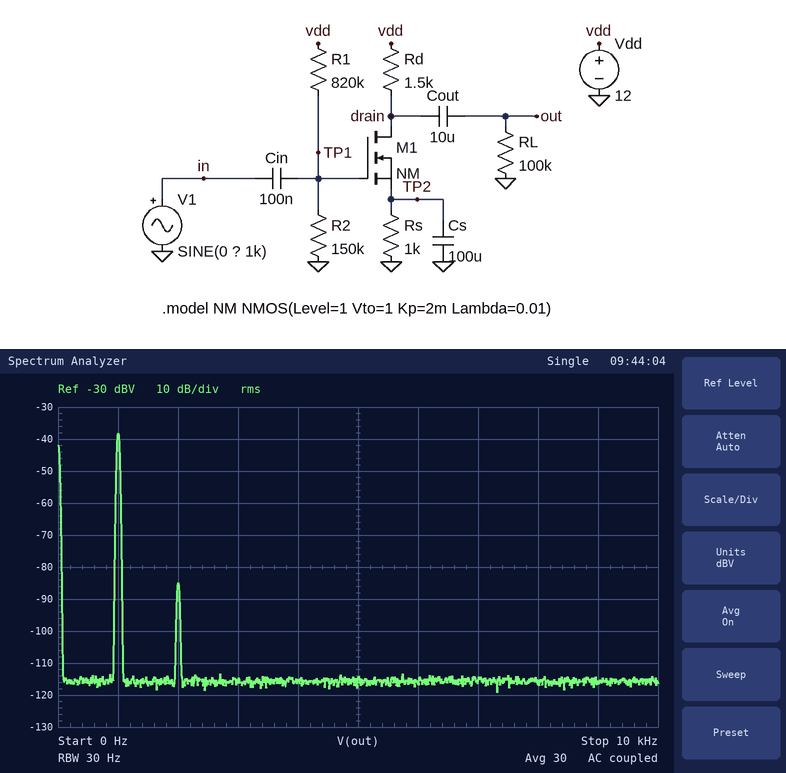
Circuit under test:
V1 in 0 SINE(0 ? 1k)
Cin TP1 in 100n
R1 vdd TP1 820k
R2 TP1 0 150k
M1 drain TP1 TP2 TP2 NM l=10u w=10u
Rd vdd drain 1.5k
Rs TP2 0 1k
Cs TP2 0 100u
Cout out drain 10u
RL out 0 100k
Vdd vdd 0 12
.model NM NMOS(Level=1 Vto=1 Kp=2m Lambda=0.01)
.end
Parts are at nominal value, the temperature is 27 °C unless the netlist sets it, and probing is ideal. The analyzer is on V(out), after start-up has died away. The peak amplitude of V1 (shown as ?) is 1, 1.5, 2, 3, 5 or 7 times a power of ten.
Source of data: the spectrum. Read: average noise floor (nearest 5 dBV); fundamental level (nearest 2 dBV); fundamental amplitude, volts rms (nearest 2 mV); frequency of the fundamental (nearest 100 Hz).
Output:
-115 dBV
-38 dBV
12 mV
1.0 kHz
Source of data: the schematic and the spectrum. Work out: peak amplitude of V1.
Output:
10 mV
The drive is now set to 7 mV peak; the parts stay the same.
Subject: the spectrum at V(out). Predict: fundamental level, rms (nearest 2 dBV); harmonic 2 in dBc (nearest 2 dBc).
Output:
-42 dBV
-50 dBc
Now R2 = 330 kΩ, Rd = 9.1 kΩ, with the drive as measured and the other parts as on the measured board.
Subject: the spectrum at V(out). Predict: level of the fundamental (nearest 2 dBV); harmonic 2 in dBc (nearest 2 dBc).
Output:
-46 dBV
-42 dBc
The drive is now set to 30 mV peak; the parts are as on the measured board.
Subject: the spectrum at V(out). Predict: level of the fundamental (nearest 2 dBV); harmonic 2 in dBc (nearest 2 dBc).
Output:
-28 dBV
-38 dBc
